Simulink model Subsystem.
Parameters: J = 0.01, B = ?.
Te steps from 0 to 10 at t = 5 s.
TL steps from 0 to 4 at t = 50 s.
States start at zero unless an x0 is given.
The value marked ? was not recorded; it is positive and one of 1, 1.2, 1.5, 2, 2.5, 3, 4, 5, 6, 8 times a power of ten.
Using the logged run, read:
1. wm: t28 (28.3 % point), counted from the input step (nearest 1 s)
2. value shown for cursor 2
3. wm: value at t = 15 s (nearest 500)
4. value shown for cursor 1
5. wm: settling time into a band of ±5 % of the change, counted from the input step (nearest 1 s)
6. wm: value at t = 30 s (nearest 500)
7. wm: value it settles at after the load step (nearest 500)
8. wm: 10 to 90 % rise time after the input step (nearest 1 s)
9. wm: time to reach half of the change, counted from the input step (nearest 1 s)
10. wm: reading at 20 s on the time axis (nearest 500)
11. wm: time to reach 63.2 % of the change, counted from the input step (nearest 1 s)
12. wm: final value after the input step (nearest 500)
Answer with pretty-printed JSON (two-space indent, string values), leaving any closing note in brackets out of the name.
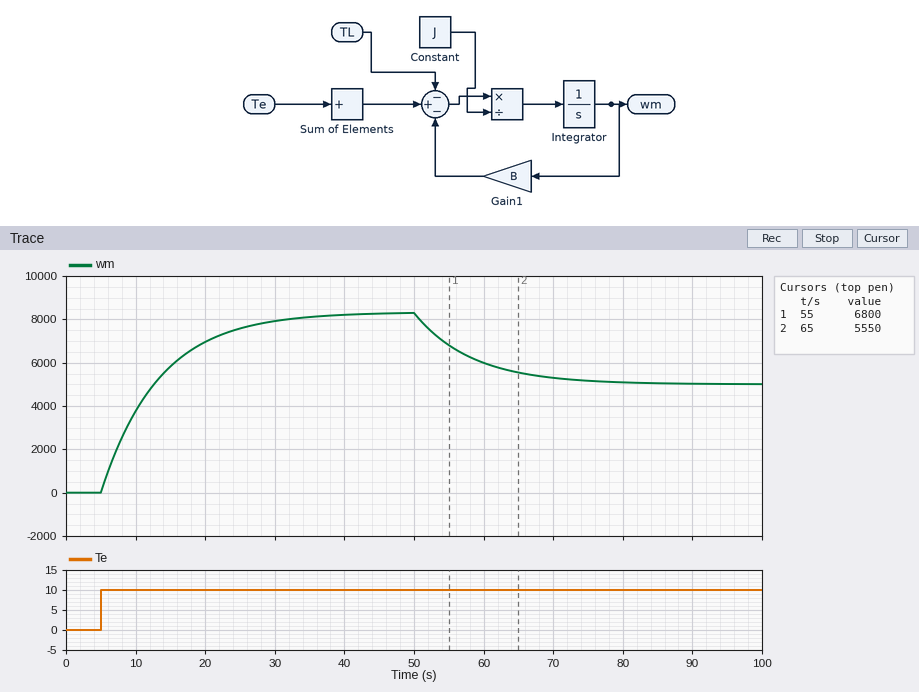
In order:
{
  "wm: t28 (28.3 % point), counted from the input step": "3 s",
  "value shown for cursor 2": "5550",
  "wm: value at t = 15 s": "6000",
  "value shown for cursor 1": "6800",
  "wm: settling time into a band of ±5 % of the change, counted from the input step": "25 s",
  "wm: value at t = 30 s": "8000",
  "wm: value it settles at after the load step": "5000",
  "wm: 10 to 90 % rise time after the input step": "18 s",
  "wm: time to reach half of the change, counted from the input step": "6 s",
  "wm: reading at 20 s on the time axis": "7000",
  "wm: time to reach 63.2 % of the change, counted from the input step": "8 s",
  "wm: final value after the input step": "8500"
}
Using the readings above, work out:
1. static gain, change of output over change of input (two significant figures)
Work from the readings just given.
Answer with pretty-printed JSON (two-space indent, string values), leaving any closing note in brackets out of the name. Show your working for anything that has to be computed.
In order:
{
  "static gain, change of output over change of input": "(8500 - 0) / (10 - 0) = 850"
}
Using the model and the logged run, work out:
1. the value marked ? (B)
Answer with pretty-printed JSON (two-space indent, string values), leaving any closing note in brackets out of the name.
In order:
{
  "the value marked ?": "0.0012"
}
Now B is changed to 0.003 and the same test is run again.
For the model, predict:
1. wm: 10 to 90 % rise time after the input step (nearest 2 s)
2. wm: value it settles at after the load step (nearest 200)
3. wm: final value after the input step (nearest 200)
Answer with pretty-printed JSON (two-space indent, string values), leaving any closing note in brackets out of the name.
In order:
{
  "wm: 10 to 90 % rise time after the input step": "8 s",
  "wm: value it settles at after the load step": "2000",
  "wm: final value after the input step": "3400"
}
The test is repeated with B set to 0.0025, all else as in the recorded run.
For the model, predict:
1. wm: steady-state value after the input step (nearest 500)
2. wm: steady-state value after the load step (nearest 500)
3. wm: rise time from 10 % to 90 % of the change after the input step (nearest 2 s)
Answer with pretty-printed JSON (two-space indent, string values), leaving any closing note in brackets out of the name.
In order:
{
  "wm: steady-state value after the input step": "4000",
  "wm: steady-state value after the load step": "2500",
  "wm: rise time from 10 % to 90 % of the change after the input step": "8 s"
}
